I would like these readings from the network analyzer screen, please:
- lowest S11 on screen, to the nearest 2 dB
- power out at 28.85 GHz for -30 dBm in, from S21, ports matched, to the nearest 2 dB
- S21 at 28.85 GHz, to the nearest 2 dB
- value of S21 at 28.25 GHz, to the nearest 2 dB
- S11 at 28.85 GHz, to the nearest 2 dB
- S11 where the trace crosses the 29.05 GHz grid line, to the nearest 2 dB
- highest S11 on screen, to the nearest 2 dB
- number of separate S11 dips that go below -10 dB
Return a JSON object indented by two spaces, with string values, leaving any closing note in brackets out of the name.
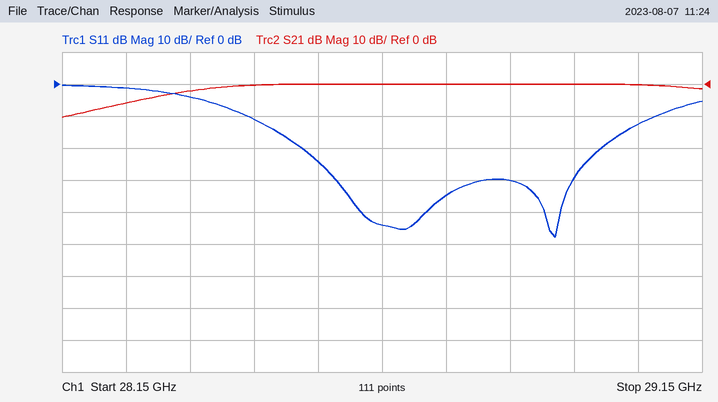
{
  "lowest S11 on screen, to the nearest 2 dB": "-48 dB",
  "power out at 28.85 GHz for -30 dBm in, from S21, ports matched, to the nearest 2 dB": "-30 dBm",
  "S21 at 28.85 GHz, to the nearest 2 dB": "0 dB",
  "value of S21 at 28.25 GHz, to the nearest 2 dB": "-6 dB",
  "S11 at 28.85 GHz, to the nearest 2 dB": "-30 dB",
  "S11 where the trace crosses the 29.05 GHz grid line, to the nearest 2 dB": "-12 dB",
  "highest S11 on screen, to the nearest 2 dB": "0 dB",
  "number of separate S11 dips that go below -10 dB": "2"
}
